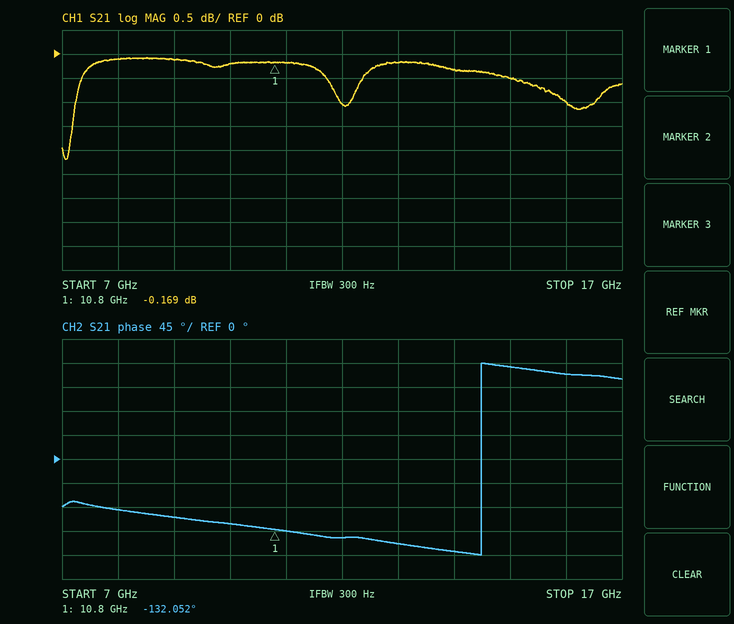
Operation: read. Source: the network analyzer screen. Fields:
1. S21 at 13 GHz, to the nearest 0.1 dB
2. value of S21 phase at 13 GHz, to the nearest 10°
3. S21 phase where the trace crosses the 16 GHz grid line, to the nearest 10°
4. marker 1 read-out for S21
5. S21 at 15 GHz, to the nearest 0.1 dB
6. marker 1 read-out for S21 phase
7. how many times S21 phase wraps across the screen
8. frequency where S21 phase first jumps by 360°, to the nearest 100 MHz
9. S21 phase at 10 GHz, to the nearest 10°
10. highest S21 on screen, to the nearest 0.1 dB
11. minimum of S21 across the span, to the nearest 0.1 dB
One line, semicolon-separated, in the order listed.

-0.2 dB; -160°; 160°; -0.169 dB; -0.5 dB; -132.052°; 1; 14.5 GHz; -120°; -0.1 dB; -2.2 dB
